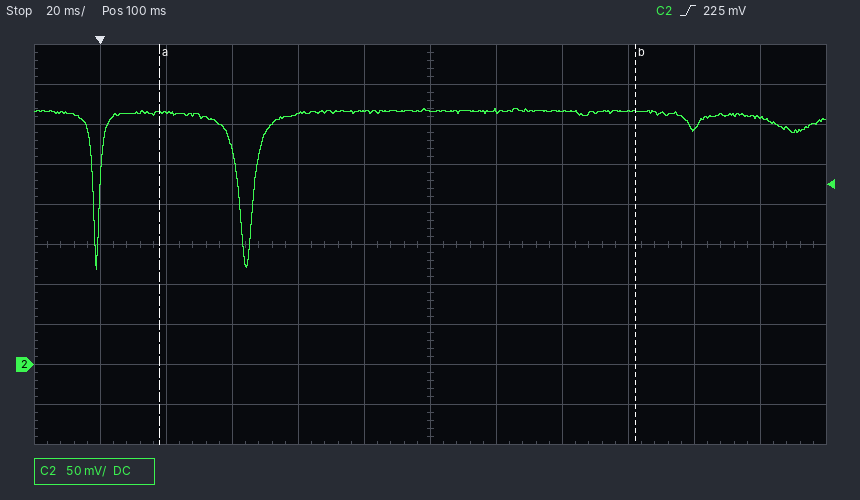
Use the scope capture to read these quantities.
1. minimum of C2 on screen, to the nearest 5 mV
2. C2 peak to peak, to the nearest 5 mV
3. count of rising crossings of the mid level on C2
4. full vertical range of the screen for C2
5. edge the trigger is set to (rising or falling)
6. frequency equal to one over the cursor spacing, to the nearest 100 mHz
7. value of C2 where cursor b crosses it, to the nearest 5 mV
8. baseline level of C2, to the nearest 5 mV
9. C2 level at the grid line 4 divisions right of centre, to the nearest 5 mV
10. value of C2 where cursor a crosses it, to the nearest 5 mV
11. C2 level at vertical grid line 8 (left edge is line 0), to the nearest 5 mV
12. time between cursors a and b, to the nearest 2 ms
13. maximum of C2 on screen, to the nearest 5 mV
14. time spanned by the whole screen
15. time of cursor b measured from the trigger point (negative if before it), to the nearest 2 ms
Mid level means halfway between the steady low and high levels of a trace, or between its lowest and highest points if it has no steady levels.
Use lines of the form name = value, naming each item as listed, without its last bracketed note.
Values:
minimum of C2 on screen, to the nearest 5 mV = 120 mV
C2 peak to peak, to the nearest 5 mV = 200 mV
count of rising crossings of the mid level on C2 = 2
full vertical range of the screen for C2 = 500 mV
edge the trigger is set to = rising
frequency equal to one over the cursor spacing, to the nearest 100 mHz = 6.9 Hz
value of C2 where cursor b crosses it, to the nearest 5 mV = 315 mV
baseline level of C2, to the nearest 5 mV = 315 mV
C2 level at the grid line 4 divisions right of centre, to the nearest 5 mV = 295 mV
value of C2 where cursor a crosses it, to the nearest 5 mV = 315 mV
C2 level at vertical grid line 8 (left edge is line 0), to the nearest 5 mV = 315 mV
time between cursors a and b, to the nearest 2 ms = 144 ms
maximum of C2 on screen, to the nearest 5 mV = 320 mV
time spanned by the whole screen = 240 ms
time of cursor b measured from the trigger point (negative if before it), to the nearest 2 ms = +162 ms
